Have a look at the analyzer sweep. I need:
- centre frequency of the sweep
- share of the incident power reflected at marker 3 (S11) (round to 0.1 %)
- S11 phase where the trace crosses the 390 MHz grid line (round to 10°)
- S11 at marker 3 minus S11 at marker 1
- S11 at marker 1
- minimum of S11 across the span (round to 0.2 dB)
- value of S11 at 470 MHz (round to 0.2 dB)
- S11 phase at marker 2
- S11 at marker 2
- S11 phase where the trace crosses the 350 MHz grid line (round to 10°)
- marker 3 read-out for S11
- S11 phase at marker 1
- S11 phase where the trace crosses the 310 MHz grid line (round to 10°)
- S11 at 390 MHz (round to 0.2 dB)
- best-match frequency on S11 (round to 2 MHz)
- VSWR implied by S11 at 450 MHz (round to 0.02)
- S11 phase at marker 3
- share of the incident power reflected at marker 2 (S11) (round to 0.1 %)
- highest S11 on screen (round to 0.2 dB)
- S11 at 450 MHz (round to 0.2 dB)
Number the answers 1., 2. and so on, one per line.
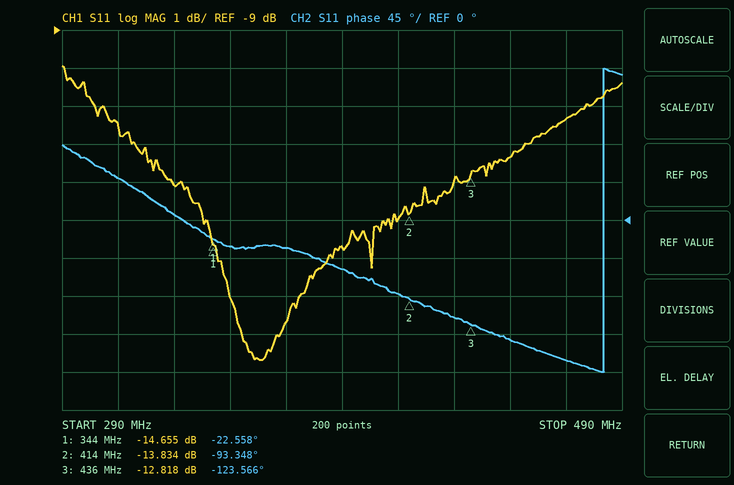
1. 390 MHz
2. 5.2 %
3. -60°
4. 1.837 dB
5. -14.655 dB
6. -17.6 dB
7. -11.4 dB
8. -93.348°
9. -13.834 dB
10. -30°
11. -12.818 dB
12. -22.558°
13. 50°
14. -14.8 dB
15. 360 MHz
16. 1.64
17. -123.566°
18. 4.1 %
19. -10.0 dB
20. -12.4 dB
